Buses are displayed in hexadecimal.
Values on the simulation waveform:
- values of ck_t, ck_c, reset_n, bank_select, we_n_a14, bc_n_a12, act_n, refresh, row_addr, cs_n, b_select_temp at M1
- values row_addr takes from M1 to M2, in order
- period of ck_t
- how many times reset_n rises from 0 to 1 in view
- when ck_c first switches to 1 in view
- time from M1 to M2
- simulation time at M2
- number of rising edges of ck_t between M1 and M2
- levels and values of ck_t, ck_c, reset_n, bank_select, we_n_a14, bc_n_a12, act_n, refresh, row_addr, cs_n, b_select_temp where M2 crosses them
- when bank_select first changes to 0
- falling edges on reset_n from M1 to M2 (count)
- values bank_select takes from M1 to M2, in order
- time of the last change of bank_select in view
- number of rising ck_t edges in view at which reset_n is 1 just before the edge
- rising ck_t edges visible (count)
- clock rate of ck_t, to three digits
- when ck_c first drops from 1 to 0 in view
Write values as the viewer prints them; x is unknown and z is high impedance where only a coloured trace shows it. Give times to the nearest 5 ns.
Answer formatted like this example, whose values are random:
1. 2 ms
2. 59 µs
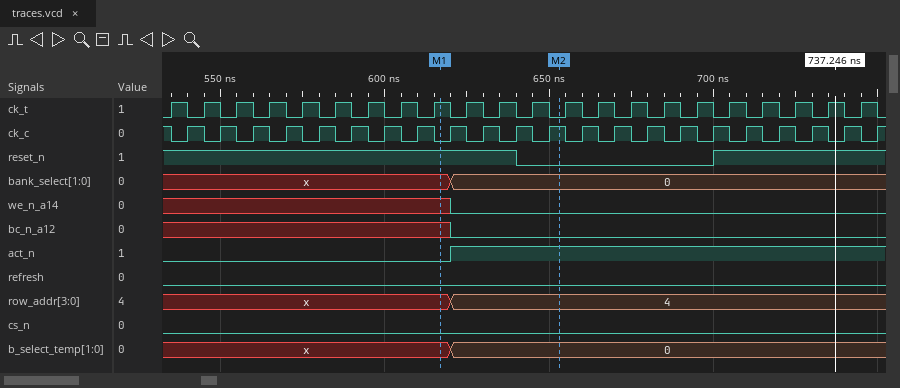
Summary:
1. ck_t=1, ck_c=0, reset_n=1, bank_select=x, we_n_a14=x, bc_n_a12=x, act_n=0, refresh=0, row_addr=x, cs_n=0, b_select_temp=x
2. x, 4
3. 10 ns
4. 1
5. 540 ns
6. 35 ns
7. 655 ns
8. 3
9. ck_t=0, ck_c=1, reset_n=0, bank_select=0, we_n_a14=0, bc_n_a12=0, act_n=1, refresh=0, row_addr=4, cs_n=0, b_select_temp=0
10. 620 ns
11. 1
12. x, 0
13. 620 ns
14. 16
15. 22
16. 100 MHz
17. 535 ns
